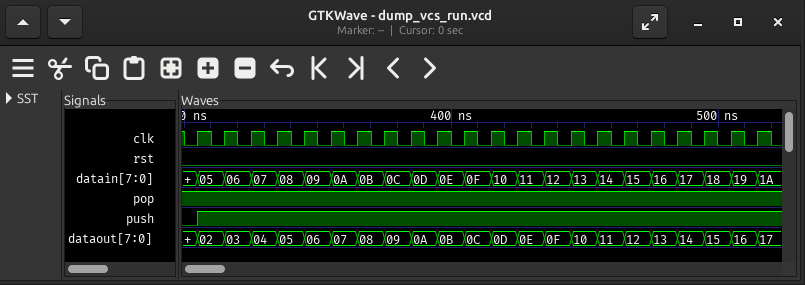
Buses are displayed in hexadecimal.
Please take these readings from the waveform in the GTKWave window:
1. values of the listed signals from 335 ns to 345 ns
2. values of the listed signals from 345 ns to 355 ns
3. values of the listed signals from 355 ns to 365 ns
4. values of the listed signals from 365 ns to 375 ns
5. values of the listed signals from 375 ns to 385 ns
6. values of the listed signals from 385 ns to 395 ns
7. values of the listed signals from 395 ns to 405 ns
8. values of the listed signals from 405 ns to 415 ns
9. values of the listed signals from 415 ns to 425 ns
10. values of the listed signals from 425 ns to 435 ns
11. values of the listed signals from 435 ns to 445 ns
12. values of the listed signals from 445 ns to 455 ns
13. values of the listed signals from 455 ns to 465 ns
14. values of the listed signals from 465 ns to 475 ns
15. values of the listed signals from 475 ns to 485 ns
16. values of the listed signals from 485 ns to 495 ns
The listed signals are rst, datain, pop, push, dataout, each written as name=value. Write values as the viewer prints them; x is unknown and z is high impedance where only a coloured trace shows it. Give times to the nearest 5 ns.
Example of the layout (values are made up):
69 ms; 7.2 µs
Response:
rst=0, datain=08, pop=1, push=1, dataout=05; rst=0, datain=09, pop=1, push=1, dataout=06; rst=0, datain=0A, pop=1, push=1, dataout=07; rst=0, datain=0B, pop=1, push=1, dataout=08; rst=0, datain=0C, pop=1, push=1, dataout=09; rst=0, datain=0D, pop=1, push=1, dataout=0A; rst=0, datain=0E, pop=1, push=1, dataout=0B; rst=0, datain=0F, pop=1, push=1, dataout=0C; rst=0, datain=10, pop=1, push=1, dataout=0D; rst=0, datain=11, pop=1, push=1, dataout=0E; rst=0, datain=12, pop=1, push=1, dataout=0F; rst=0, datain=13, pop=1, push=1, dataout=10; rst=0, datain=14, pop=1, push=1, dataout=11; rst=0, datain=15, pop=1, push=1, dataout=12; rst=0, datain=16, pop=1, push=1, dataout=13; rst=0, datain=17, pop=1, push=1, dataout=14
